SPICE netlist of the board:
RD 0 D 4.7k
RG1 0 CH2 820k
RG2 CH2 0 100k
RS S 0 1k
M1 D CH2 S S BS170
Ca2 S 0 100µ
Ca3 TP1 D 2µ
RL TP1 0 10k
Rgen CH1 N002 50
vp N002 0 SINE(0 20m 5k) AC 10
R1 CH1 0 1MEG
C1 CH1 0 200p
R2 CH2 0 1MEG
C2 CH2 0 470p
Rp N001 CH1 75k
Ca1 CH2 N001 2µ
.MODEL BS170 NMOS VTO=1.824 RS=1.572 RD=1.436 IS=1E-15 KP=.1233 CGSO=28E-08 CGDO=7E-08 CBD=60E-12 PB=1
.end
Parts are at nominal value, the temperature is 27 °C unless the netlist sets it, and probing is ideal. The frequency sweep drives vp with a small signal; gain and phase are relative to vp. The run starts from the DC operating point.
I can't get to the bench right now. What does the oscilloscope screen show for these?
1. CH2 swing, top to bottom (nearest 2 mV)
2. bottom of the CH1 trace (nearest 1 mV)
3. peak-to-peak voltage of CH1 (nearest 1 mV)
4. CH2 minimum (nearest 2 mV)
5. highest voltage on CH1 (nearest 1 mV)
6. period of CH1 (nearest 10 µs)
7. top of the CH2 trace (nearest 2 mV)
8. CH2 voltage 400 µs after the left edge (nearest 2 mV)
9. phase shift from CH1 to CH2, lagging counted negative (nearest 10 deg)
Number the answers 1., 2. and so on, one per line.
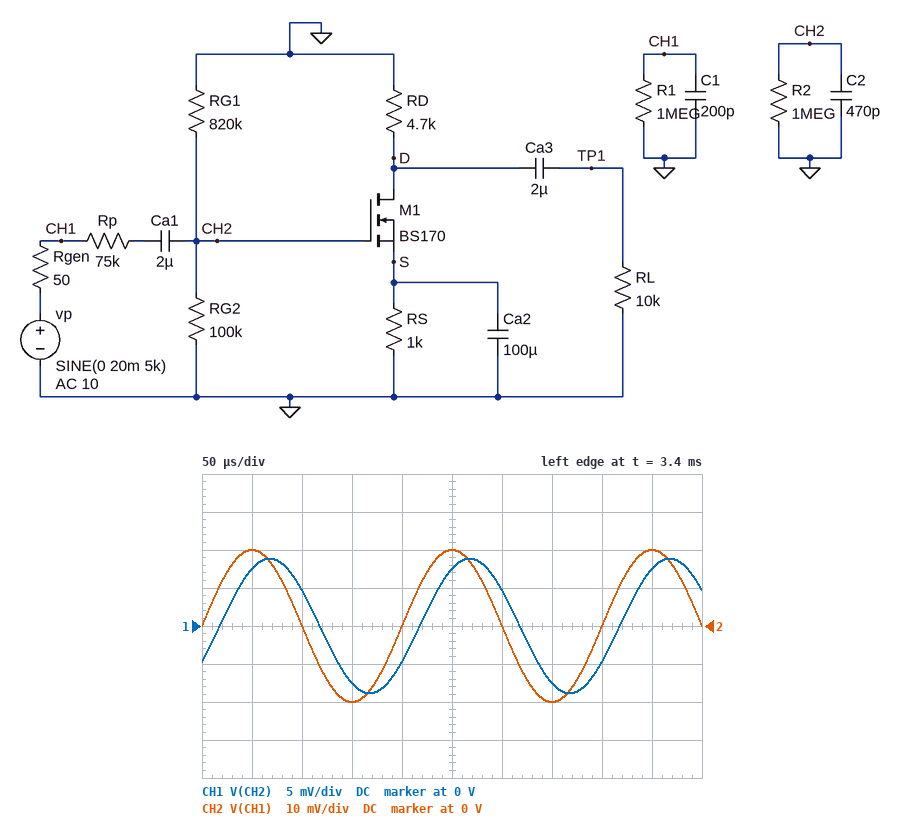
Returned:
1. 40 mV
2. -9 mV
3. 18 mV
4. -20 mV
5. 9 mV
6. 200 µs
7. 20 mV
8. 0 V
9. 30 deg
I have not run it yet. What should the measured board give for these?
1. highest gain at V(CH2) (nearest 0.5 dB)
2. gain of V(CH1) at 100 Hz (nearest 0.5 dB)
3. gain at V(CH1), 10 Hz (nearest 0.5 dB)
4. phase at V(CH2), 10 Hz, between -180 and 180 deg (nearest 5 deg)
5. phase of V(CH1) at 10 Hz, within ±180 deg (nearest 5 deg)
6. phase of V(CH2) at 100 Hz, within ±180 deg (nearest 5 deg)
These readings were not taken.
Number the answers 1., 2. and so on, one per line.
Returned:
1. -5.5 dB
2. 0 dB
3. 0 dB
4. 5 deg
5. 0 deg
6. 0 deg
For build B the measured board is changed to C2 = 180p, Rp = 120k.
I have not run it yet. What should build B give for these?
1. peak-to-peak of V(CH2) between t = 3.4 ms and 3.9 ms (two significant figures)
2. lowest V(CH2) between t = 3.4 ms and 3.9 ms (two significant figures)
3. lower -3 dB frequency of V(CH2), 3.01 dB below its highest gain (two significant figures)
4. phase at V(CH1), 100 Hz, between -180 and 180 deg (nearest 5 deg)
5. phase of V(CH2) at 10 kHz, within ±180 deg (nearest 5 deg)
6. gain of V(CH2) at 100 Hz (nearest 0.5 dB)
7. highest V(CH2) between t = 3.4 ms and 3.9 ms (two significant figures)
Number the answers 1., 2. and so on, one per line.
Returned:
1. 15 mV
2. -7.7 mV
3. 390 mHz
4. 0 deg
5. -35 deg
6. -8.0 dB
7. 7.7 mV
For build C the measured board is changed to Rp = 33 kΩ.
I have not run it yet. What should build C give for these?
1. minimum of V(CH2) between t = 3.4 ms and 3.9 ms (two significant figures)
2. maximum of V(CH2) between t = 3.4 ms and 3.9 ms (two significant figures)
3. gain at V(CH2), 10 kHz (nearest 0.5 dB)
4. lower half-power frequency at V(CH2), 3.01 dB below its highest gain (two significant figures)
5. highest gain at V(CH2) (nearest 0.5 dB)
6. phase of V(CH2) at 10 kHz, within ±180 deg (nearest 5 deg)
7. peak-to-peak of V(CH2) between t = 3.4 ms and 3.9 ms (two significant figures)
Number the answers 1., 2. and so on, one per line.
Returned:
1. -13 mV
2. 13 mV
3. -5.0 dB
4. 690 mHz
5. -3.0 dB
6. -35 deg
7. 27 mV
